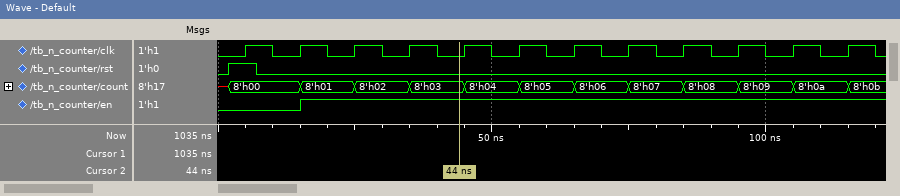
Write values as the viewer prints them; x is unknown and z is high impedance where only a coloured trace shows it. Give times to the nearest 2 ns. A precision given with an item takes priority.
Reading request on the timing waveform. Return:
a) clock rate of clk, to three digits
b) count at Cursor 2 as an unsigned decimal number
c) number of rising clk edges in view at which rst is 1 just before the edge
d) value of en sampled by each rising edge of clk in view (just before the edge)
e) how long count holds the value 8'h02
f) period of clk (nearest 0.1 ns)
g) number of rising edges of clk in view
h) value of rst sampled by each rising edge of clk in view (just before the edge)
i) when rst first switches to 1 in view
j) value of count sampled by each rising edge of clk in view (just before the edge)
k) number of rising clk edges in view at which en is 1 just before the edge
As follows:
100 MHz
3
1
0 0 1 1 1 1 1 1 1 1 1 1
10 ns
10 ns
12
1 0 0 0 0 0 0 0 0 0 0 0
2 ns
8'h00, 8'h00, 8'h01, 8'h02, 8'h03, 8'h04, 8'h05, 8'h06, 8'h07, 8'h08, 8'h09, 8'h0a
10
